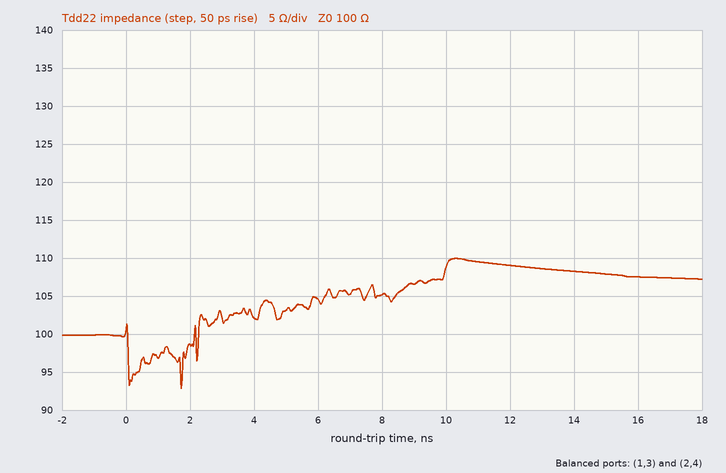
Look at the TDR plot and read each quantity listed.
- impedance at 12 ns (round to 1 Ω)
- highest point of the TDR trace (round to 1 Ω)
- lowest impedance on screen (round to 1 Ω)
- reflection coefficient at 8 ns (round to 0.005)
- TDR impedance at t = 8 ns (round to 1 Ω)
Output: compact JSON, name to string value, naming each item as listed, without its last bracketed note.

{"impedance at 12 ns": "109 Ω", "highest point of the TDR trace": "110 Ω", "lowest impedance on screen": "93 Ω", "reflection coefficient at 8 ns": "+0.025", "TDR impedance at t = 8 ns": "105 Ω"}
